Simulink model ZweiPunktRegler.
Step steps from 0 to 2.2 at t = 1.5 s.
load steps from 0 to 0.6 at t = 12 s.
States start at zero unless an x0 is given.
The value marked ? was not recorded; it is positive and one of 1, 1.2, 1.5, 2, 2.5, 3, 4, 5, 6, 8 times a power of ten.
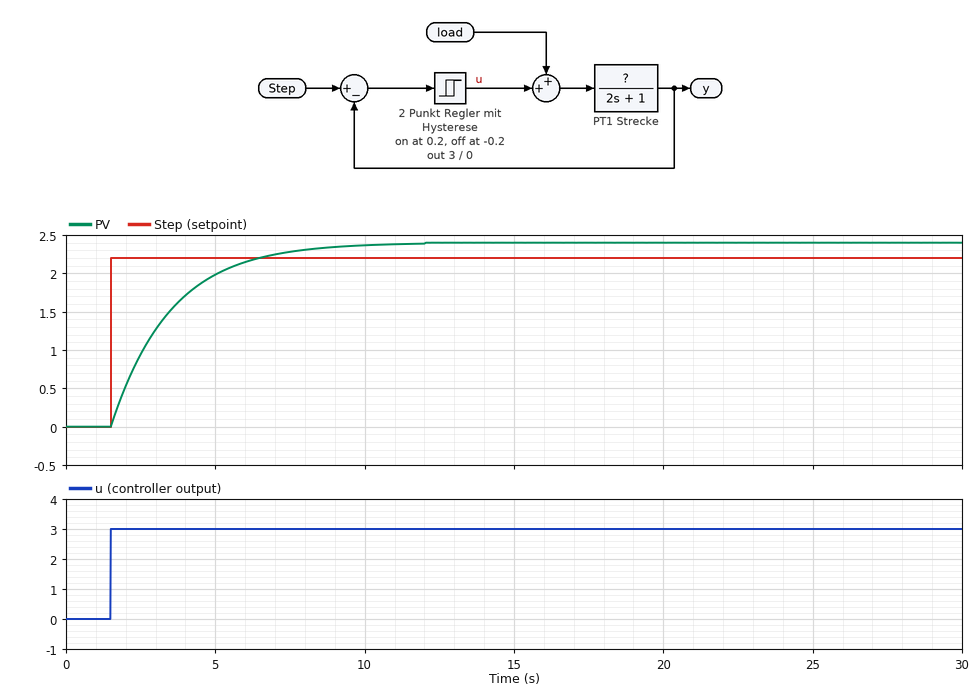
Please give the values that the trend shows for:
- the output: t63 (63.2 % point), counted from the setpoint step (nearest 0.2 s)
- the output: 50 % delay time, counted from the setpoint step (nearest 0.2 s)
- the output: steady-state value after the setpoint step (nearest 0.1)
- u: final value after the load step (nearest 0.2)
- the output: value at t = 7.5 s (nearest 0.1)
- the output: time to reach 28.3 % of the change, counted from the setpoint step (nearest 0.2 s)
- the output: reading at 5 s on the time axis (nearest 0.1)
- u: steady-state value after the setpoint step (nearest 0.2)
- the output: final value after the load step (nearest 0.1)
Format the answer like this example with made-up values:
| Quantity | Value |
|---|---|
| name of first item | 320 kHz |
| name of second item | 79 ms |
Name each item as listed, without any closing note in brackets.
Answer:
| Quantity | Value |
|---|---|
| the output: t63 (63.2 % point), counted from the setpoint step | 2.0 s |
| the output: 50 % delay time, counted from the setpoint step | 1.4 s |
| the output: steady-state value after the setpoint step | 2.4 |
| u: final value after the load step | 3.0 |
| the output: value at t = 7.5 s | 2.3 |
| the output: time to reach 28.3 % of the change, counted from the setpoint step | 0.6 s |
| the output: reading at 5 s on the time axis | 2.0 |
| u: steady-state value after the setpoint step | 3.0 |
| the output: final value after the load step | 2.4 |
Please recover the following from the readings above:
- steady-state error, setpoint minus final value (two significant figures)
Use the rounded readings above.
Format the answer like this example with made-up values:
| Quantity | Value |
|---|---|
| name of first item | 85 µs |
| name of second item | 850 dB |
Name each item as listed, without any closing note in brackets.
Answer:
| Quantity | Value |
|---|---|
| steady-state error, setpoint minus final value | -0.20 |
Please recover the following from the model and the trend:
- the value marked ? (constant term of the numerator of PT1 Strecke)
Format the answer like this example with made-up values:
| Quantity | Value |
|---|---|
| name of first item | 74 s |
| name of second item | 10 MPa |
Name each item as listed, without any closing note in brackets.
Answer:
| Quantity | Value |
|---|---|
| the value marked ? | 0.8 |
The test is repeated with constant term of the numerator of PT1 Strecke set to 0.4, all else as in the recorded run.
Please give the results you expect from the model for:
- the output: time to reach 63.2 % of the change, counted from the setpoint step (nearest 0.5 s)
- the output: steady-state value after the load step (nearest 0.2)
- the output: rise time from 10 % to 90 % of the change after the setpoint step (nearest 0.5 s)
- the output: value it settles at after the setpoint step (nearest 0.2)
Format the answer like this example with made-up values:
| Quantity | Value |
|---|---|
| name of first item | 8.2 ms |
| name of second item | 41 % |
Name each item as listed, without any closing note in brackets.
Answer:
| Quantity | Value |
|---|---|
| the output: time to reach 63.2 % of the change, counted from the setpoint step | 2.0 s |
| the output: steady-state value after the load step | 1.4 |
| the output: rise time from 10 % to 90 % of the change after the setpoint step | 4.5 s |
| the output: value it settles at after the setpoint step | 1.2 |
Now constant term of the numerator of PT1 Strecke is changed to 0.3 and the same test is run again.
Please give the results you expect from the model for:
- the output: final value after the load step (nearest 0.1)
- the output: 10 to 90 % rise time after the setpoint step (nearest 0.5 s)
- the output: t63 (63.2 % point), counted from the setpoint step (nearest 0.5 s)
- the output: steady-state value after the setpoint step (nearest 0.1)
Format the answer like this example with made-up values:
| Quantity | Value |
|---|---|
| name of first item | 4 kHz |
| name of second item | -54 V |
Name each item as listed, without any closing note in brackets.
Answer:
| Quantity | Value |
|---|---|
| the output: final value after the load step | 1.1 |
| the output: 10 to 90 % rise time after the setpoint step | 4.5 s |
| the output: t63 (63.2 % point), counted from the setpoint step | 2.0 s |
| the output: steady-state value after the setpoint step | 0.9 |
